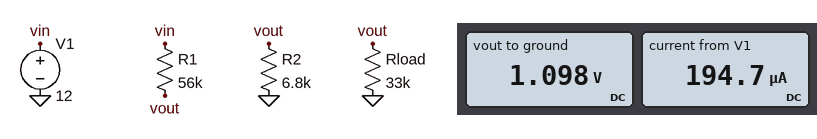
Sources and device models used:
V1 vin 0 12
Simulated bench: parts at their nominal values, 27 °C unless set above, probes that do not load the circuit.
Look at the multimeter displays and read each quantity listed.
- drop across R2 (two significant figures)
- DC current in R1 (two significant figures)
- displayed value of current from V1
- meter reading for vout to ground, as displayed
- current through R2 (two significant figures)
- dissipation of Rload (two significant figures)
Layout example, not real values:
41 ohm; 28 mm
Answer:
1.1 V; 190 µA; 194.7 µA; 1.098 V; 160 µA; 37 µW
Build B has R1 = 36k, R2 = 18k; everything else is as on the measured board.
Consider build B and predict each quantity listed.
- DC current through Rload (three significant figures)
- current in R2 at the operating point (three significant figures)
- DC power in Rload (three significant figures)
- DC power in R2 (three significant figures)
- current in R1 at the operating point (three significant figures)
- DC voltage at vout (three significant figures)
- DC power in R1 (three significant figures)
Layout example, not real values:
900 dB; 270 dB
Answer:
88.9 µA; 163 µA; 261 µW; 478 µW; 252 µA; 2.93 V; 2.28 mW
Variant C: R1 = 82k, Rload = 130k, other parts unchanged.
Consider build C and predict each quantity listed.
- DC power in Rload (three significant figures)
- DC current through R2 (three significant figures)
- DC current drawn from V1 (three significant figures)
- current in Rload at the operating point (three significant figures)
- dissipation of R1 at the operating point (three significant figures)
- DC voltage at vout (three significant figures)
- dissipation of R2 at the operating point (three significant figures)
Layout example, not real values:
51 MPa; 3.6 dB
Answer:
5.91 µW; 129 µA; 136 µA; 6.74 µA; 1.51 mW; 877 mV; 113 µW
